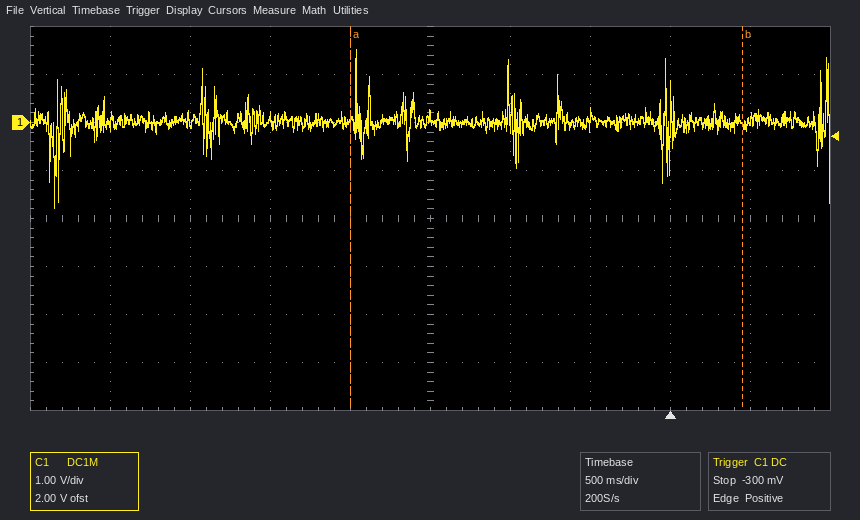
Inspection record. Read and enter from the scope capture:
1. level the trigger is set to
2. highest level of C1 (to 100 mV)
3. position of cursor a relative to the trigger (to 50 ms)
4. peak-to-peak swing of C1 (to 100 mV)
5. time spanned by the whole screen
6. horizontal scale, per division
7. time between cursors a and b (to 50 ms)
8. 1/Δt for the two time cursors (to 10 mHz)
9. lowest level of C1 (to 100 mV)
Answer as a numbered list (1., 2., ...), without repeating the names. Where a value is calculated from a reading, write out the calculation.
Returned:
1. -300 mV
2. 1.5 V
3. -2.00 s
4. 1.5 V − (-1.8 V) = 3.3 V
5. 5 s
6. 500 ms
7. 2.45 s
8. 1 / 2.45 s ≈ 410 mHz
9. -1.8 V
